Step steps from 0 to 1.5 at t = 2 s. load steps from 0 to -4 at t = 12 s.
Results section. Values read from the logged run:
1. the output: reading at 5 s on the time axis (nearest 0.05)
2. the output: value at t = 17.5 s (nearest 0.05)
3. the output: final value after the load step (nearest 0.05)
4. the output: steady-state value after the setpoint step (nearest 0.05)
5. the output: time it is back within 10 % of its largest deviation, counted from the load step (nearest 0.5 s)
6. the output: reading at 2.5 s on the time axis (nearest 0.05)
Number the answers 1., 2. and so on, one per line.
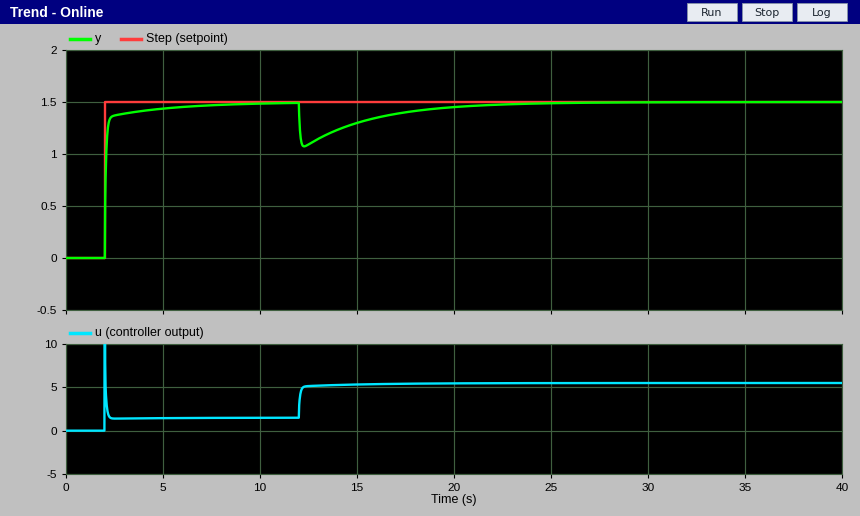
1. 1.45
2. 1.40
3. 1.50
4. 1.50
5. 8.5 s
6. 1.35
